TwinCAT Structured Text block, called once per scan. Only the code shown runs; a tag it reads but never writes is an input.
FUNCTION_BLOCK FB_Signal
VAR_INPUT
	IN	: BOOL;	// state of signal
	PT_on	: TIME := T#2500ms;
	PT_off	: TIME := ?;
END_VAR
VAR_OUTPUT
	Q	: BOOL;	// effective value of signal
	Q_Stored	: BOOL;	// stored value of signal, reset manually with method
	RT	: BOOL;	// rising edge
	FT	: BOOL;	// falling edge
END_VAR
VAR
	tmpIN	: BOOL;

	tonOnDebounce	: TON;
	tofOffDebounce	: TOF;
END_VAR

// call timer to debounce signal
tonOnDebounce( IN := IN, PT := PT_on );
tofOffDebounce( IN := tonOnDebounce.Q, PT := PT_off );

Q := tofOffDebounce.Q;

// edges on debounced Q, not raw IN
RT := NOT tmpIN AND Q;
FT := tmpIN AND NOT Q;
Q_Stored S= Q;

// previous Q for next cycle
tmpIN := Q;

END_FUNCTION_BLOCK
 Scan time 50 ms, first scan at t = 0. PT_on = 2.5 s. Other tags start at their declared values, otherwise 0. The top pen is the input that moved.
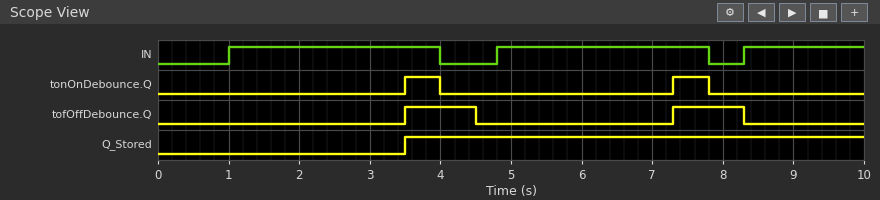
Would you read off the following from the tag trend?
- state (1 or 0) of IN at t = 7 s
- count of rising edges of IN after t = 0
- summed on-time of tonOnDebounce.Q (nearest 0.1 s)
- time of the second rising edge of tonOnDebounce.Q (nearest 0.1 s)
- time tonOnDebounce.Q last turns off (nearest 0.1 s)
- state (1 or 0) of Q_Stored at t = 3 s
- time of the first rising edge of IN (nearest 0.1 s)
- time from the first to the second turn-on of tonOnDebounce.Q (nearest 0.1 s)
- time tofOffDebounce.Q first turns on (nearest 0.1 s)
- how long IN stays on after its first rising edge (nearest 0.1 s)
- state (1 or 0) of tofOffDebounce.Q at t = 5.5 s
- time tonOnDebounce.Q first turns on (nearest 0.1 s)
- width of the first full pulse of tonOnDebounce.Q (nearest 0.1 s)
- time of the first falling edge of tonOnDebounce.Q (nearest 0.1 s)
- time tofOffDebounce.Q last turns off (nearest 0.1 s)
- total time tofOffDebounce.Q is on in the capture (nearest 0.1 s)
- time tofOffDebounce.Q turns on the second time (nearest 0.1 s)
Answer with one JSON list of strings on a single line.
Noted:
["1", "3", "1.0 s", "7.3 s", "7.8 s", "0", "1.0 s", "3.8 s", "3.5 s", "3.0 s", "0", "3.5 s", "0.5 s", "4.0 s", "8.3 s", "2.0 s", "7.3 s"]
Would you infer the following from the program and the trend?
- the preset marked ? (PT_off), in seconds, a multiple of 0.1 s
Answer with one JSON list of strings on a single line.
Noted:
["0.5 s"]
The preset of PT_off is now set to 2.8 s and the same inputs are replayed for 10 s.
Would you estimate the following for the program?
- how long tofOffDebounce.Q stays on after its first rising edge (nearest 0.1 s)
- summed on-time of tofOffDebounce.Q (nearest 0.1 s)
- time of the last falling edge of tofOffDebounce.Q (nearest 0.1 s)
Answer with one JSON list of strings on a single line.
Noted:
["3.3 s", "6.0 s", "6.8 s"]
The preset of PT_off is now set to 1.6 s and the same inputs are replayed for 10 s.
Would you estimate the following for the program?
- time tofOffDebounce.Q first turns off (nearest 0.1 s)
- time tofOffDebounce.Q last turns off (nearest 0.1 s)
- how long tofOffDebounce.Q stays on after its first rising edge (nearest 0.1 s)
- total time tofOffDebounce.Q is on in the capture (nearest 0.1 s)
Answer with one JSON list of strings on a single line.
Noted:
["5.6 s", "9.4 s", "2.1 s", "4.2 s"]
